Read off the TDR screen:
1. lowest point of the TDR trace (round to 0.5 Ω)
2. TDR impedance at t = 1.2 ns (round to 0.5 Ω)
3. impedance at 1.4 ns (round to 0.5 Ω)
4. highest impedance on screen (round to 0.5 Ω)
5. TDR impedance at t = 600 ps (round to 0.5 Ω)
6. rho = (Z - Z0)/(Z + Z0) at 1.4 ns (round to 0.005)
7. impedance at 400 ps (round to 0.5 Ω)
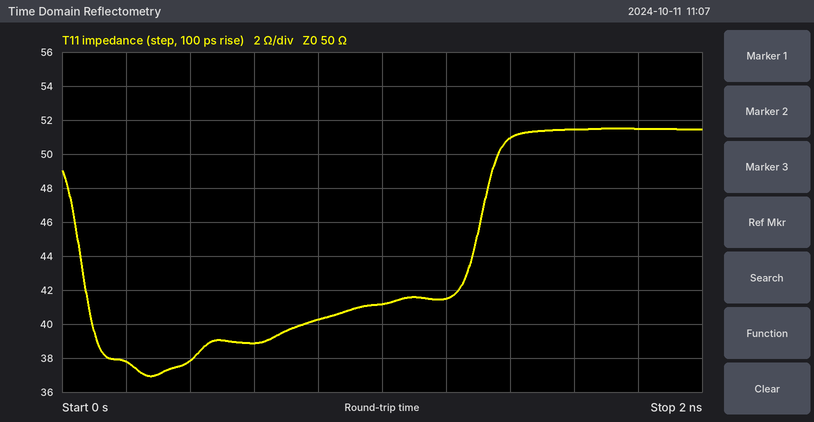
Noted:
37.0 Ω
41.5 Ω
51.0 Ω
51.5 Ω
39.0 Ω
+0.010
38.0 Ω
